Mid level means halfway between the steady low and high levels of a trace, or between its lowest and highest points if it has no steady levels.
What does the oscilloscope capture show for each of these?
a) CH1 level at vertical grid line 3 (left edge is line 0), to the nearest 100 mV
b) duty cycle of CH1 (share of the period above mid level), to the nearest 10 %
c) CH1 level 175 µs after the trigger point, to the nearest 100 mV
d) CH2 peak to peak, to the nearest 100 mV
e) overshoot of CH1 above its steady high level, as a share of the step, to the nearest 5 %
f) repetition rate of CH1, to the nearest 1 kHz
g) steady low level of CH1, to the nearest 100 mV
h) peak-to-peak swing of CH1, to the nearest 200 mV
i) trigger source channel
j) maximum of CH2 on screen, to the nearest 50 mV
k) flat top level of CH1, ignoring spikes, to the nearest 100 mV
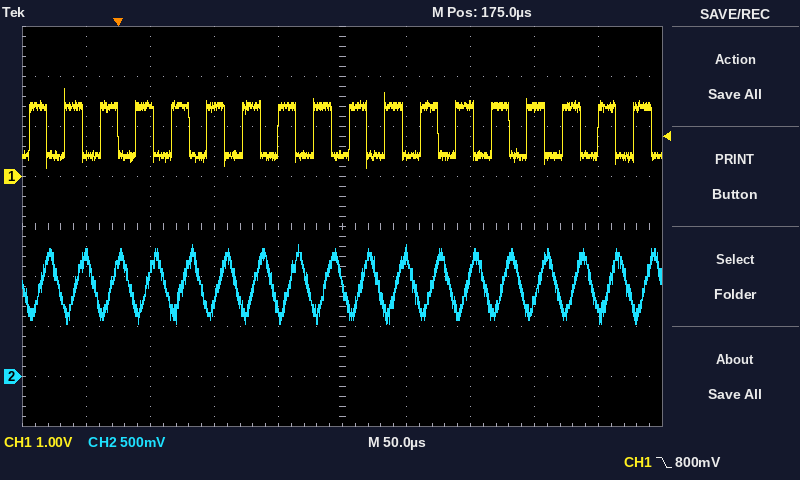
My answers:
1.4 V
50 %
400 mV
800 mV
35 %
36 kHz
400 mV
1.6 V
CH1
1.30 V
1.4 V
